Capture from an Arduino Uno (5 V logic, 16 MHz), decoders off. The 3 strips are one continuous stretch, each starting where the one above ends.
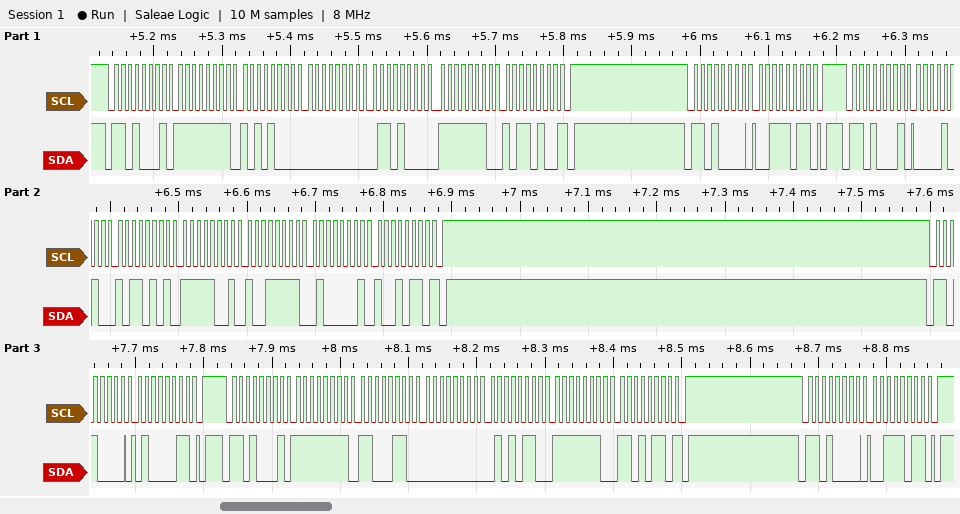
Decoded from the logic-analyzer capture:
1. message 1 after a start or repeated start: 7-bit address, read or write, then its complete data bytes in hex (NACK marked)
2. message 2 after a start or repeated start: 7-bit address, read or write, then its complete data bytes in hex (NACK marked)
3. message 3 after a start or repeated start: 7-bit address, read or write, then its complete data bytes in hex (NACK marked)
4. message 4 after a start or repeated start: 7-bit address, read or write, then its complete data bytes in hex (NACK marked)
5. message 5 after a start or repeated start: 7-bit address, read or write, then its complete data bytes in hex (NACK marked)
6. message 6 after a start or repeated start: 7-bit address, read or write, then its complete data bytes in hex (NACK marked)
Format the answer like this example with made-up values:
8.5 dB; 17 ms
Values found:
0x68 read: FF A8 00 68 FE B4 NACK; 0x68 write: 3B; 0x68 read: 0A B5 F9 9F 41 96 NACK; 0x68 write: 43; 0x68 read: FF C6 00 56 FE D6 NACK; 0x68 write: 3B
